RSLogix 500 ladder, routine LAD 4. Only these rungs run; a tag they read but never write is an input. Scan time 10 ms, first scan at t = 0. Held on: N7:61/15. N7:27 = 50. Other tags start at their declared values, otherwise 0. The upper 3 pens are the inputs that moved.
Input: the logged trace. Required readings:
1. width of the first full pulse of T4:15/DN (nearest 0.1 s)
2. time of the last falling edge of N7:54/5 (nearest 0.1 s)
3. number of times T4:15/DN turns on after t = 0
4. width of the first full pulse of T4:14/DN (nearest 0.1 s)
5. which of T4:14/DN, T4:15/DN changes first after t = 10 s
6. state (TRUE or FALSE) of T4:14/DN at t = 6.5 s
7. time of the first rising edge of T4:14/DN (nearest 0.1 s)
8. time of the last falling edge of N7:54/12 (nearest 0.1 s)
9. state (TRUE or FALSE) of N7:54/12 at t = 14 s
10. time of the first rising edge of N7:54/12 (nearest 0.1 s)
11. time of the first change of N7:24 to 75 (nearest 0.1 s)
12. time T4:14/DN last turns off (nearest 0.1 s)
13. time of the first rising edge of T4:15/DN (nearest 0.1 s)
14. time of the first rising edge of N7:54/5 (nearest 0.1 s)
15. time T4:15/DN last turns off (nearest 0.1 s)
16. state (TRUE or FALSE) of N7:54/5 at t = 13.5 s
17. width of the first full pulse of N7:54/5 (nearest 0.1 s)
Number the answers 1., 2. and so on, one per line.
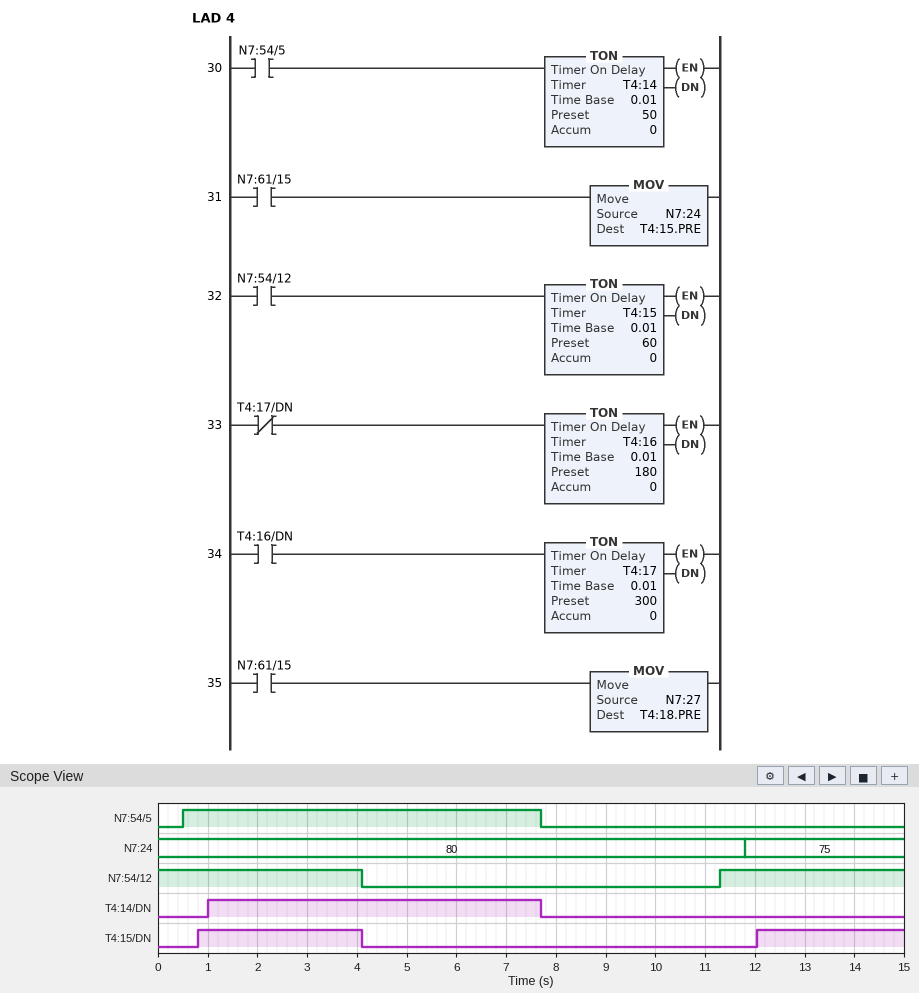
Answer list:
1. 3.3 s
2. 7.7 s
3. 2
4. 6.7 s
5. T4:15/DN
6. TRUE
7. 1.0 s
8. 4.1 s
9. TRUE
10. 11.3 s
11. 11.8 s
12. 7.7 s
13. 0.8 s
14. 0.5 s
15. 4.1 s
16. FALSE
17. 7.2 s
